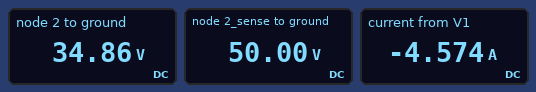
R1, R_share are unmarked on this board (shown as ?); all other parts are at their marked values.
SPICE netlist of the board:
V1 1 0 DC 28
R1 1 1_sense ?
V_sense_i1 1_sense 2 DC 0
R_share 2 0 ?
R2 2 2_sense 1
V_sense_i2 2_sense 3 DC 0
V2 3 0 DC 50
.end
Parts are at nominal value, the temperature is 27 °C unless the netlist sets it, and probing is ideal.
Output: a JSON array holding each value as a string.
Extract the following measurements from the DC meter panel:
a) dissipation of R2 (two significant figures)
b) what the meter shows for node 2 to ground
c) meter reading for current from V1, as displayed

["230 W", "34.86 V", "-4.574 A"]
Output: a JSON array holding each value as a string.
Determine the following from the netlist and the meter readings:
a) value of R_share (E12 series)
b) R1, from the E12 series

["3.3 Ω", "1.5 Ω"]
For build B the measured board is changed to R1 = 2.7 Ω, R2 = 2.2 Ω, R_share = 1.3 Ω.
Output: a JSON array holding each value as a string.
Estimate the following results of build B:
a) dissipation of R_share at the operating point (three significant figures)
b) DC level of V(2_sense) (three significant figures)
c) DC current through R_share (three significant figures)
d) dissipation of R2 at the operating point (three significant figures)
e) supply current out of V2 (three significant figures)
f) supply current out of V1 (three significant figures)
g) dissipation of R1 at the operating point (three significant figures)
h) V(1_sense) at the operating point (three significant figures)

["332 W", "50.0 V", "16.0 A", "389 W", "13.3 A", "2.68 A", "19.4 W", "20.8 V"]
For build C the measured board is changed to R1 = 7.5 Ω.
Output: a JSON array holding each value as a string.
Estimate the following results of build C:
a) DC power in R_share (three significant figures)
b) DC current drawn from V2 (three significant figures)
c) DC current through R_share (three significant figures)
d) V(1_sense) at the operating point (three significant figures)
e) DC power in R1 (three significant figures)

["424 W", "12.6 A", "11.3 A", "37.4 V", "11.8 W"]
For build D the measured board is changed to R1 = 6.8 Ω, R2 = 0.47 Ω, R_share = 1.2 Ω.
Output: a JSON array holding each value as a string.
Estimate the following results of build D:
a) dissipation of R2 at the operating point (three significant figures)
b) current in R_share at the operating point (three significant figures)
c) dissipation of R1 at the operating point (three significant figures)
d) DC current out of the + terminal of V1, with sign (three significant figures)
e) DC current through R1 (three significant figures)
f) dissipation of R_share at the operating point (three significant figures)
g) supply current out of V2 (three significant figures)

["444 W", "29.6 A", "8.39 W", "-1.11 A", "1.11 A", "1.05 kW", "30.7 A"]
